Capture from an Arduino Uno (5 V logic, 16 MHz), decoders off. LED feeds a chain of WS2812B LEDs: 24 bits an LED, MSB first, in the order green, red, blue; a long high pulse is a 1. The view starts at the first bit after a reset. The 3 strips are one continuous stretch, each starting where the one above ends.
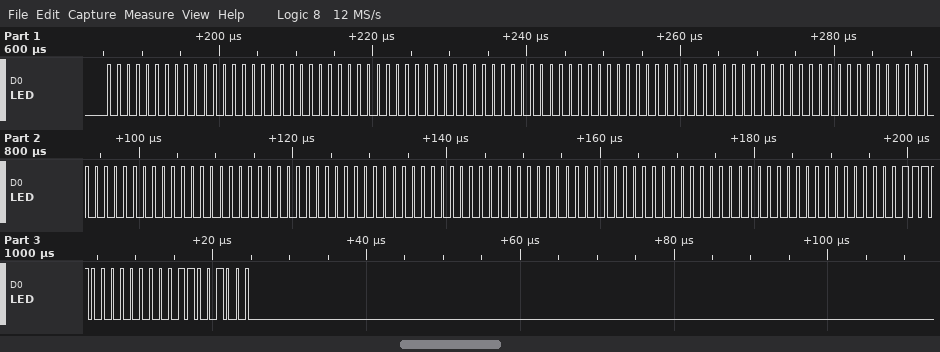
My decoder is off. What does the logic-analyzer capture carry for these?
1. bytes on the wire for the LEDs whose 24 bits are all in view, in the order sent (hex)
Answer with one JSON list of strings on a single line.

["00 00 00 00 00 00 00 00 00 00 00 00 00 00 00 00 00 00 00 00 00 1E 00 C8"]
